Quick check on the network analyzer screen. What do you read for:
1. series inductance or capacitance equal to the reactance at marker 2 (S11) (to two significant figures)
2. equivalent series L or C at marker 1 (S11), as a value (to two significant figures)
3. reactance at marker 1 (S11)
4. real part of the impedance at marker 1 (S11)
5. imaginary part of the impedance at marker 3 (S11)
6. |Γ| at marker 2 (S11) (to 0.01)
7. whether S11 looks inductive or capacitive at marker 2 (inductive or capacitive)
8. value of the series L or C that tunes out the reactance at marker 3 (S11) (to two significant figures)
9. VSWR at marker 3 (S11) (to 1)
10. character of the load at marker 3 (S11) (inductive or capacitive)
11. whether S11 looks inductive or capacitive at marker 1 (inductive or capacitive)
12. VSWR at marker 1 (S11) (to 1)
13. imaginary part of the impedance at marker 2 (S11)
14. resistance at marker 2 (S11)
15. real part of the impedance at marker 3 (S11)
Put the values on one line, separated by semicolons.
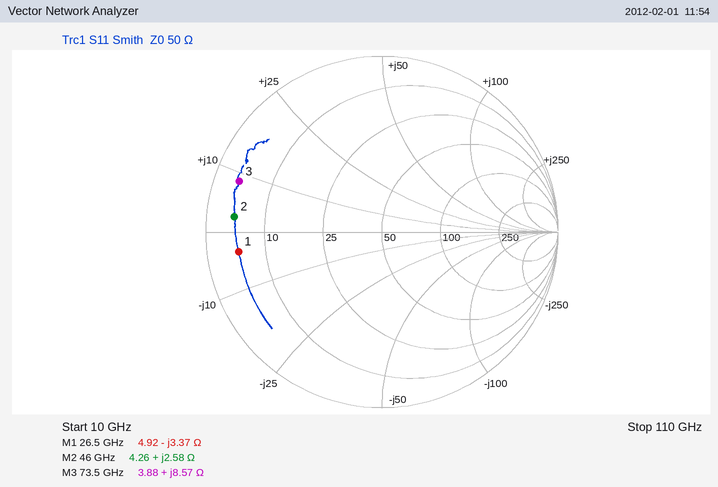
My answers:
8.9 pH; 1.8 pF; -3.37 Ω; 4.92 Ω; +8.57 Ω; 0.84; inductive; 250 fF; 13; inductive; capacitive; 10; +2.58 Ω; 4.26 Ω; 3.88 Ω
